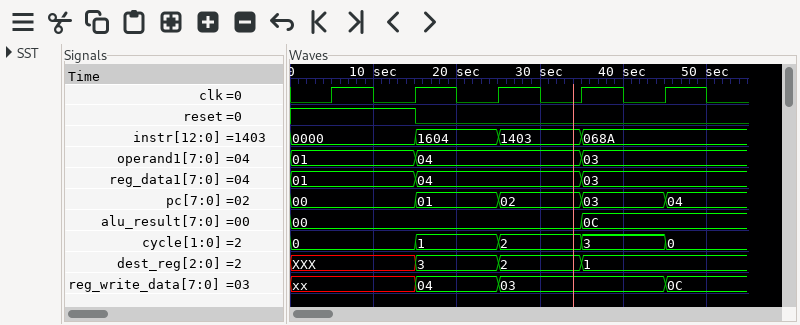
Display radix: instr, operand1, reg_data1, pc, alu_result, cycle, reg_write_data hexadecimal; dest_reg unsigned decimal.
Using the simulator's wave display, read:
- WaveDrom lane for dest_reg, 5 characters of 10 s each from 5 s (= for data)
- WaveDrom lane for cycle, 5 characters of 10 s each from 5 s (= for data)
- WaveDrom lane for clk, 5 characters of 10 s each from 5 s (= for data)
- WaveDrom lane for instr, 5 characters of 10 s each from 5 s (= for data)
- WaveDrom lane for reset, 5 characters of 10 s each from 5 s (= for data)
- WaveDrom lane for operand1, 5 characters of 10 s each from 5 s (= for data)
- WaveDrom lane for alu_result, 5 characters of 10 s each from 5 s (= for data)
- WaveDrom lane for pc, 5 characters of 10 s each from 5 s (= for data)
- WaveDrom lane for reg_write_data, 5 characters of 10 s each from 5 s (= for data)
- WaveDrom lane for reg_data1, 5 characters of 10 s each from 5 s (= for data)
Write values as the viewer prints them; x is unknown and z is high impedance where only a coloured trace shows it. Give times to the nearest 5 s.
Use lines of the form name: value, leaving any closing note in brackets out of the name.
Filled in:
WaveDrom lane for dest_reg, 5 characters of 10 s each from 5 s: {name: 'dest_reg', wave: 'x===.', data: '3 2 1'}
WaveDrom lane for cycle, 5 characters of 10 s each from 5 s: {name: 'cycle', wave: '=====', data: '0 1 2 3 0'}
WaveDrom lane for clk, 5 characters of 10 s each from 5 s: {name: 'clk', wave: 'p....'}
WaveDrom lane for instr, 5 characters of 10 s each from 5 s: {name: 'instr', wave: '====.', data: '0000 1604 1403 068A'}
WaveDrom lane for reset, 5 characters of 10 s each from 5 s: {name: 'reset', wave: '10...'}
WaveDrom lane for operand1, 5 characters of 10 s each from 5 s: {name: 'operand1', wave: '==.=.', data: '01 04 03'}
WaveDrom lane for alu_result, 5 characters of 10 s each from 5 s: {name: 'alu_result', wave: '=..=.', data: '00 0C'}
WaveDrom lane for pc, 5 characters of 10 s each from 5 s: {name: 'pc', wave: '=====', data: '00 01 02 03 04'}
WaveDrom lane for reg_write_data, 5 characters of 10 s each from 5 s: {name: 'reg_write_data', wave: 'x==.=', data: '04 03 0C'}
WaveDrom lane for reg_data1, 5 characters of 10 s each from 5 s: {name: 'reg_data1', wave: '==.=.', data: '01 04 03'}
